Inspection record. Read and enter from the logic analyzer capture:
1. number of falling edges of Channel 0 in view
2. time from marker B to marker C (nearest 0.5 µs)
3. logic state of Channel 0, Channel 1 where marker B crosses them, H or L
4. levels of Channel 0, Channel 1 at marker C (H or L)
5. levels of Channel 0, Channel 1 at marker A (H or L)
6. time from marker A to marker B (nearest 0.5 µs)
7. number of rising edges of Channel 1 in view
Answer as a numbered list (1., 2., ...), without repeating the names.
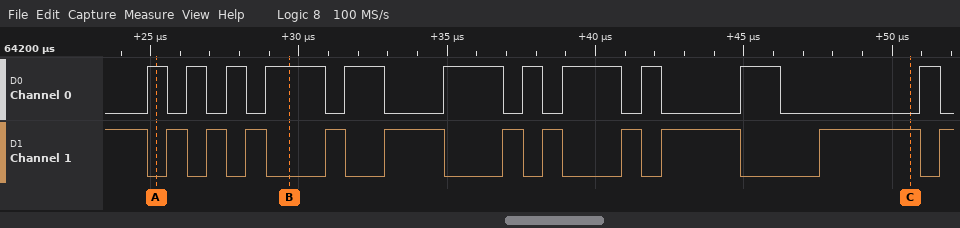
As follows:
1. 11
2. 21 µs
3. Channel 0=H, Channel 1=L
4. Channel 0=L, Channel 1=H
5. Channel 0=H, Channel 1=L
6. 4.5 µs
7. 11
